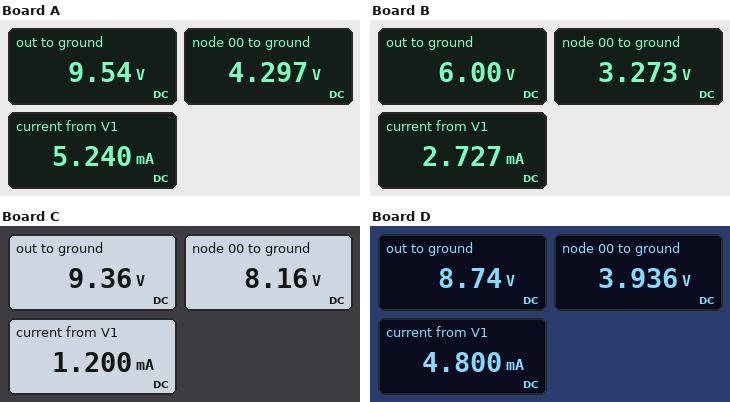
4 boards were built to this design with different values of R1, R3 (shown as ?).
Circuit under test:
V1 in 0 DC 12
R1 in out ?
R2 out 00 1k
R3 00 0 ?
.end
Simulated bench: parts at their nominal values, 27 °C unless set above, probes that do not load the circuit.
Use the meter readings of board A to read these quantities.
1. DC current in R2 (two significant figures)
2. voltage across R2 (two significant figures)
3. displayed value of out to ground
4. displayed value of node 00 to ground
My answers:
5.2 mA
5.2 V
9.54 V
4.297 V
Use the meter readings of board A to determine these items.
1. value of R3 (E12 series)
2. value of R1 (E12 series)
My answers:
820 Ω
470 Ω
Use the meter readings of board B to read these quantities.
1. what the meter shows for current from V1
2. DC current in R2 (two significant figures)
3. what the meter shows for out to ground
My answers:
2.727 mA
2.7 mA
6.00 V
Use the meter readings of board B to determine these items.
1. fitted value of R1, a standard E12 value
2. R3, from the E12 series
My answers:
2.2 kΩ
1.2 kΩ
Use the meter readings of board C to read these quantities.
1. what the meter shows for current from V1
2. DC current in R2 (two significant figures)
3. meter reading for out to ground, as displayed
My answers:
1.200 mA
1.2 mA
9.36 V
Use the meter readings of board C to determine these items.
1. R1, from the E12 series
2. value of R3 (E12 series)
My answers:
2.2 kΩ
6.8 kΩ
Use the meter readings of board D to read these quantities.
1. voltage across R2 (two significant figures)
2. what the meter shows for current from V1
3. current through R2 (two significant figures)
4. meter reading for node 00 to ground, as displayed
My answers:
4.8 V
4.800 mA
4.8 mA
3.936 V
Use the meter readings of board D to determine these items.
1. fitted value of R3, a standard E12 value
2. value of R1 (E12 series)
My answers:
820 Ω
680 Ω
